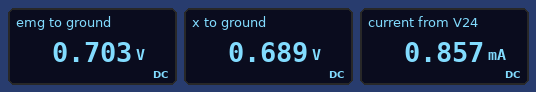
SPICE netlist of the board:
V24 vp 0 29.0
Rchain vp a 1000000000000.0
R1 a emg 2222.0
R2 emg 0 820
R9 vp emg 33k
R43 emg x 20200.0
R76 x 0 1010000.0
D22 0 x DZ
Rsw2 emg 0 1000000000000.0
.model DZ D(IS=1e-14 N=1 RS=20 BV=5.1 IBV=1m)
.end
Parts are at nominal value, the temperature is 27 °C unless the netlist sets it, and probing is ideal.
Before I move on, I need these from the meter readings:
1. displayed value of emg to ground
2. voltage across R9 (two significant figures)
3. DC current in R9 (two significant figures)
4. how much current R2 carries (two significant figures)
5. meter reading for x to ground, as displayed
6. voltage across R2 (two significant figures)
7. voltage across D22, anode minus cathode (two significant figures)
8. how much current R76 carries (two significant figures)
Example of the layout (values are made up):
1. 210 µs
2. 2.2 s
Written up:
1. 0.703 V
2. 28 V
3. 860 µA
4. 860 µA
5. 0.689 V
6. 700 mV
7. -690 mV
8. 680 nA
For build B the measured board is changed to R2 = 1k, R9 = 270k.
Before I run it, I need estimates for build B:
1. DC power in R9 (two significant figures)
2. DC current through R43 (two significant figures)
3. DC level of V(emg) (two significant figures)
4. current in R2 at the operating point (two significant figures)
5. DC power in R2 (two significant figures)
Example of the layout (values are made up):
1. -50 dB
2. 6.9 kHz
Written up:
1. 3.1 mW
2. 100 nA
3. 110 mV
4. 110 µA
5. 11 µW
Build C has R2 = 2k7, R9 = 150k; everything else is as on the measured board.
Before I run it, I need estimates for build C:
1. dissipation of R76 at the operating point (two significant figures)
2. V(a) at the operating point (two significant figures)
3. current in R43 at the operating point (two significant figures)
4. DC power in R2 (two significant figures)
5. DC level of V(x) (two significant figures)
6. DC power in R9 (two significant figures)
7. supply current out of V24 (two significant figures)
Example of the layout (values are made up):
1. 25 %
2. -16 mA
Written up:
1. 250 nW
2. 510 mV
3. 500 nA
4. 97 µW
5. 500 mV
6. 5.4 mW
7. 190 µA
